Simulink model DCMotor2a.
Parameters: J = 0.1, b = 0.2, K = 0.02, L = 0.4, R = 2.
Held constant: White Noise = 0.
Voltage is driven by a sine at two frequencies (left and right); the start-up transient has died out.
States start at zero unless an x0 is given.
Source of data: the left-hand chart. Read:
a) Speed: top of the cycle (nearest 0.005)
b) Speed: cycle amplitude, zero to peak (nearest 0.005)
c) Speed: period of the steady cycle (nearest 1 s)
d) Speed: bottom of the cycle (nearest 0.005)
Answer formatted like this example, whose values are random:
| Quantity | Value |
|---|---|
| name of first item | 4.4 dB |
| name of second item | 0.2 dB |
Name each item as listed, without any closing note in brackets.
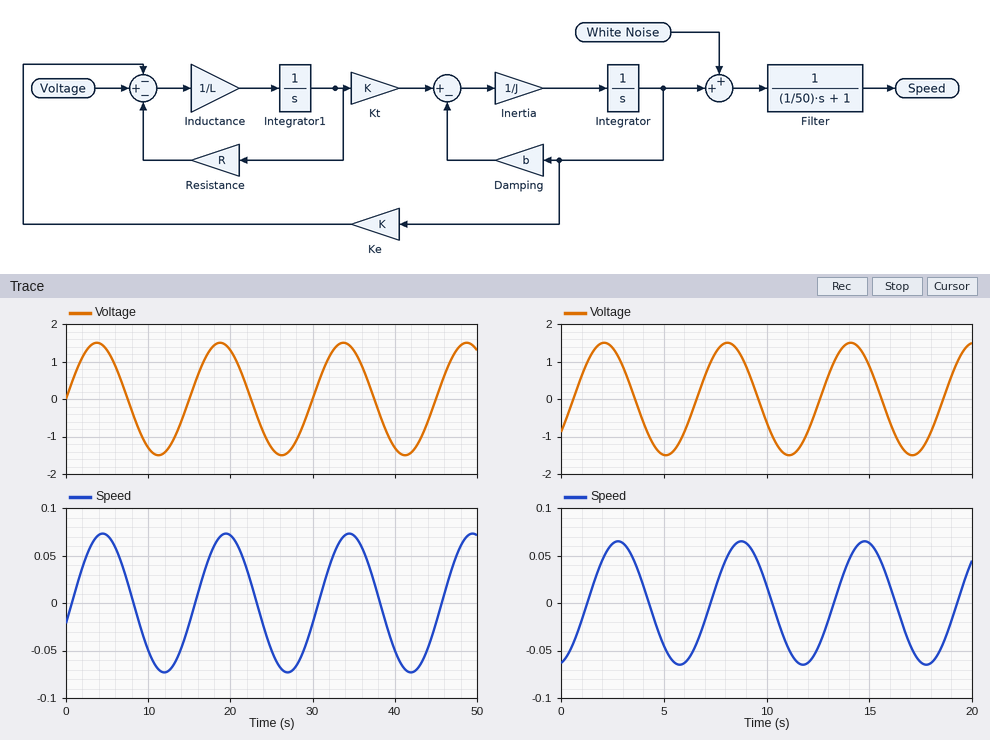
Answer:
| Quantity | Value |
|---|---|
| Speed: top of the cycle | 0.075 |
| Speed: cycle amplitude, zero to peak | 0.075 |
| Speed: period of the steady cycle | 15 s |
| Speed: bottom of the cycle | -0.075 |
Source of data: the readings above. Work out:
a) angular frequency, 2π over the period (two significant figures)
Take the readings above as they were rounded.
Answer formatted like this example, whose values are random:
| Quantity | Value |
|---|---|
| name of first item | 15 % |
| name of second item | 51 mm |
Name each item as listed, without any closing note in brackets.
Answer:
| Quantity | Value |
|---|---|
| angular frequency, 2π over the period | 0.42 rad/s |
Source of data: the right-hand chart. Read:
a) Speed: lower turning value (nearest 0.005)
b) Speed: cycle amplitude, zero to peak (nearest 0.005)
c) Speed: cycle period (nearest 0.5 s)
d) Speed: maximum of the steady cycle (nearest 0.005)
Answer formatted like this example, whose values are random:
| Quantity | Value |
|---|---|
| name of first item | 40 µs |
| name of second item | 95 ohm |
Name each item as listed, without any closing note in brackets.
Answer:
| Quantity | Value |
|---|---|
| Speed: lower turning value | -0.065 |
| Speed: cycle amplitude, zero to peak | 0.065 |
| Speed: cycle period | 6.0 s |
| Speed: maximum of the steady cycle | 0.065 |
